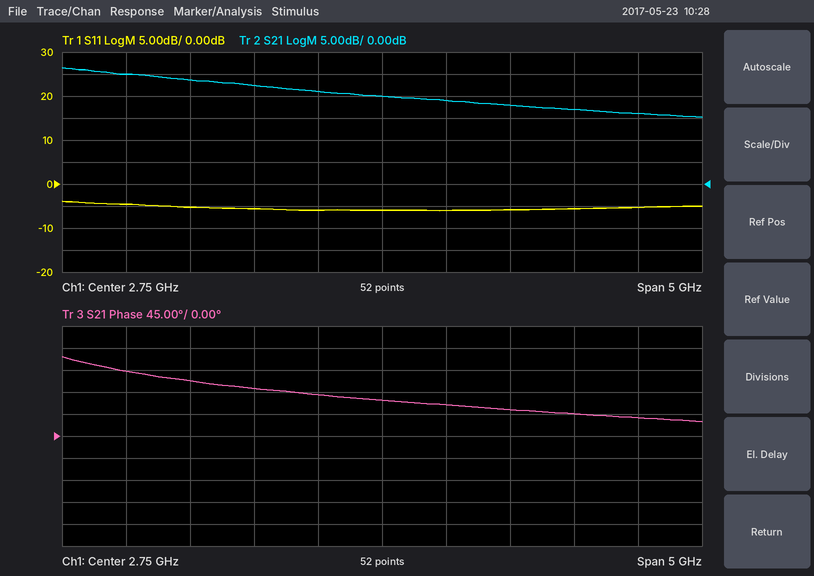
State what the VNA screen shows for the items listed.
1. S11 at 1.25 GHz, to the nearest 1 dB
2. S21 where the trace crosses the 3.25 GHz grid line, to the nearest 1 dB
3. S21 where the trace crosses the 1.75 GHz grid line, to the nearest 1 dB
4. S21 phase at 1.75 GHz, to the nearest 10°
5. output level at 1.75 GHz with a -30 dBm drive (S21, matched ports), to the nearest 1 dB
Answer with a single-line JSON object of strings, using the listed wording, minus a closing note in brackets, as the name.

{"S11 at 1.25 GHz, to the nearest 1 dB": "-5 dB", "S21 where the trace crosses the 3.25 GHz grid line, to the nearest 1 dB": "19 dB", "S21 where the trace crosses the 1.75 GHz grid line, to the nearest 1 dB": "22 dB", "S21 phase at 1.75 GHz, to the nearest 10°": "100°", "output level at 1.75 GHz with a -30 dBm drive (S21, matched ports), to the nearest 1 dB": "-8 dBm"}
